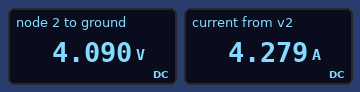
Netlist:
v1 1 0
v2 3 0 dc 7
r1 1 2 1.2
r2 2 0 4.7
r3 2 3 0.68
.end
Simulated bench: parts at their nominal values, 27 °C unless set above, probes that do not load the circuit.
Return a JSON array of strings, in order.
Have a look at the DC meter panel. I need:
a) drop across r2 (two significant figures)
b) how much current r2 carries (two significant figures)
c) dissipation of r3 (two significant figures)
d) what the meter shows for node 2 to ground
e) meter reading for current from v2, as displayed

["4.1 V", "870 mA", "12 W", "4.090 V", "4.279 A"]
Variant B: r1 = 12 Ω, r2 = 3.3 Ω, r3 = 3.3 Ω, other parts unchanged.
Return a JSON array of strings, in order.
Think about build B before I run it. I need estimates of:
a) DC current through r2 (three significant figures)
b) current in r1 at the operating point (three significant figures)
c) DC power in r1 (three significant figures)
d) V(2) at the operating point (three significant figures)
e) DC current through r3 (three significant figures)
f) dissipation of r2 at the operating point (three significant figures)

["932 mA", "256 mA", "789 mW", "3.08 V", "1.19 A", "2.87 W"]
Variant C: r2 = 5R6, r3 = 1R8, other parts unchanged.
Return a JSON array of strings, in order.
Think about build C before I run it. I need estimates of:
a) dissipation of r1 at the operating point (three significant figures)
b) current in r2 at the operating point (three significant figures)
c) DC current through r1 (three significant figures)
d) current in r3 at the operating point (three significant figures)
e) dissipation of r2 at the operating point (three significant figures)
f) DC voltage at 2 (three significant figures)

["5.13 W", "443 mA", "2.07 A", "2.51 A", "1.10 W", "2.48 V"]
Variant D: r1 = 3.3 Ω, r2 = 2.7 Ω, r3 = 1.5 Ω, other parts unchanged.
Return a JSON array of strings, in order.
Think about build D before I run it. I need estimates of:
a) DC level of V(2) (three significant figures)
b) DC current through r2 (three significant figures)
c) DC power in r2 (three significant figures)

["3.48 V", "1.29 A", "4.49 W"]
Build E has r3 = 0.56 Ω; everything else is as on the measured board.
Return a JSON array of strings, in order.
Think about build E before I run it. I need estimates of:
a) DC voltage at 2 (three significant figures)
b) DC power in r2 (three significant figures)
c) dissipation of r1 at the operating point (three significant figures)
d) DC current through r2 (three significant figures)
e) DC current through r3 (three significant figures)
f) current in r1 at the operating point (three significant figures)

["4.41 V", "4.15 W", "16.2 W", "939 mA", "4.62 A", "3.68 A"]
